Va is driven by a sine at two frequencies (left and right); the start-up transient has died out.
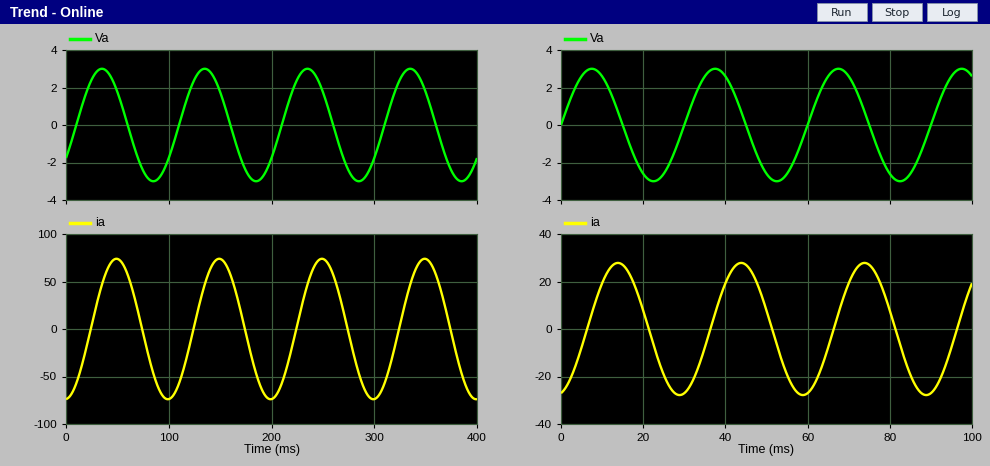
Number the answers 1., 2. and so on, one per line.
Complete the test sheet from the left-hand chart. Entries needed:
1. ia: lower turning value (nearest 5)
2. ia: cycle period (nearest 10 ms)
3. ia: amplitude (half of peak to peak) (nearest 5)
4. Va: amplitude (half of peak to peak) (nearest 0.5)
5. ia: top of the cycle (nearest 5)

1. -75
2. 100 ms
3. 75
4. 3.0
5. 75
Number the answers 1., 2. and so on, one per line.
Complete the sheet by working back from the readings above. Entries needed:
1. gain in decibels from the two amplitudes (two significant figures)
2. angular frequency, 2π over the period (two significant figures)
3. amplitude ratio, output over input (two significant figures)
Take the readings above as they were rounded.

1. 28 dB
2. 0.063 rad/ms
3. 25
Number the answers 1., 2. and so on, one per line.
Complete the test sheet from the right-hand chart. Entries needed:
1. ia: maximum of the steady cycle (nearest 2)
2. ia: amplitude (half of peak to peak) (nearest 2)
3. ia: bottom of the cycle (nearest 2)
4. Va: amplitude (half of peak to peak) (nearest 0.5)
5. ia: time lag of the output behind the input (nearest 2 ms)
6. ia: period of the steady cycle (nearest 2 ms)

1. 28
2. 28
3. -28
4. 3.0
5. 6 ms
6. 30 ms
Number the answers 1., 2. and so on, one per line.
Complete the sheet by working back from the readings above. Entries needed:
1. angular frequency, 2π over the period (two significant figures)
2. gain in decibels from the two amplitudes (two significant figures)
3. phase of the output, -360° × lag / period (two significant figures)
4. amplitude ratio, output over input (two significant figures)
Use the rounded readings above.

1. 0.21 rad/ms
2. 19 dB
3. -72°
4. 9.3
